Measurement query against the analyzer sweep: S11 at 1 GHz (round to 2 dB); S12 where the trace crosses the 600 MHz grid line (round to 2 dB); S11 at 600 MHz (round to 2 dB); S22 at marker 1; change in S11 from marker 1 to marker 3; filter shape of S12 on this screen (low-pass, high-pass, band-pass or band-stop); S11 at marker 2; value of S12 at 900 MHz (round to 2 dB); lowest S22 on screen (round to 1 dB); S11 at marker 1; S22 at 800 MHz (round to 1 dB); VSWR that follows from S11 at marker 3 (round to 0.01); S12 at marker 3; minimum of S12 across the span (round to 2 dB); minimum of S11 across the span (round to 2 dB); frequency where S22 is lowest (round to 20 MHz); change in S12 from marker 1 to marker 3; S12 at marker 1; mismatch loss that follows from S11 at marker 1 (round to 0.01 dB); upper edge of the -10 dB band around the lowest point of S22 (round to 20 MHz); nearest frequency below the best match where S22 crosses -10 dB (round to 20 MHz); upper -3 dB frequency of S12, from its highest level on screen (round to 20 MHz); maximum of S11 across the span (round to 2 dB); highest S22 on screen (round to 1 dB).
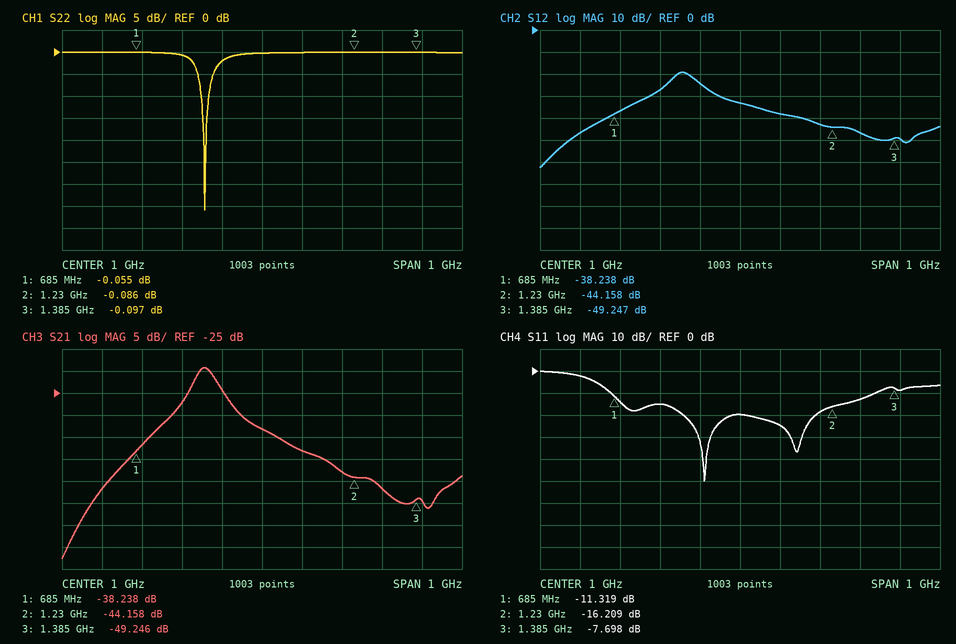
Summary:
-20 dB
-46 dB
-2 dB
-0.055 dB
3.621 dB
band-pass
-16.209 dB
-24 dB
-36 dB
-11.319 dB
-1 dB
2.40
-49.247 dB
-62 dB
-50 dB
860 MHz
-11.009 dB
-38.238 dB
0.33 dB
860 MHz
840 MHz
880 MHz
0 dB
0 dB
